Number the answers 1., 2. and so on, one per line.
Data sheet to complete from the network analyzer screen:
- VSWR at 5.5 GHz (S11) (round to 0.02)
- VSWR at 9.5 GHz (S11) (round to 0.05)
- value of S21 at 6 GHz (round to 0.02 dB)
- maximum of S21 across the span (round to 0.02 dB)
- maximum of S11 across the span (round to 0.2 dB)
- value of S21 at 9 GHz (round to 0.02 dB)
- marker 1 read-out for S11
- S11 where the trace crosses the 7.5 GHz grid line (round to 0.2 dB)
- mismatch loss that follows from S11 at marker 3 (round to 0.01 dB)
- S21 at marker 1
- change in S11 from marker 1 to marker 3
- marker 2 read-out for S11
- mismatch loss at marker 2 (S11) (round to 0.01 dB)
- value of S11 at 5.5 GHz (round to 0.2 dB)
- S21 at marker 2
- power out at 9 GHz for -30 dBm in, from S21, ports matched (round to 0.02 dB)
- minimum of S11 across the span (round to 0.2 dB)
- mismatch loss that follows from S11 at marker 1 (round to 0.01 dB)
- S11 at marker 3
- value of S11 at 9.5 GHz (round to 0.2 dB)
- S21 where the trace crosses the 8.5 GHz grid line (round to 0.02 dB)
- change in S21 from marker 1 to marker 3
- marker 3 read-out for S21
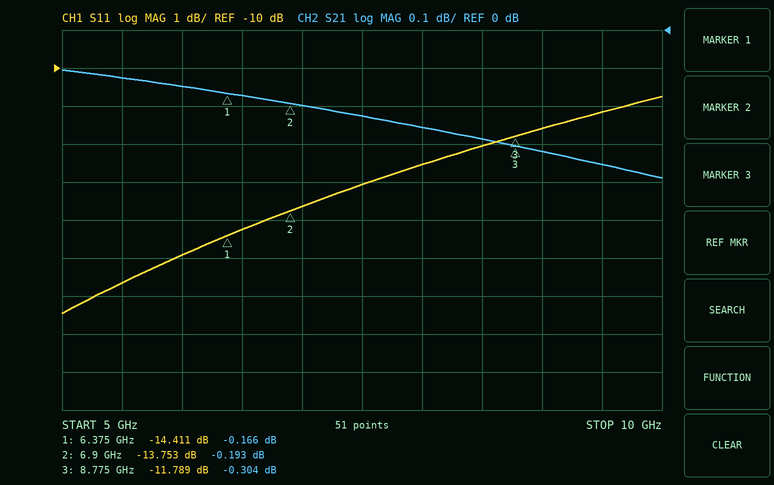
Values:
1. 1.40
2. 1.75
3. -0.14 dB
4. -0.10 dB
5. -10.8 dB
6. -0.32 dB
7. -14.411 dB
8. -13.0 dB
9. 0.30 dB
10. -0.166 dB
11. 2.622 dB
12. -13.753 dB
13. 0.19 dB
14. -15.6 dB
15. -0.193 dB
16. -30.32 dBm
17. -16.4 dB
18. 0.16 dB
19. -11.789 dB
20. -11.2 dB
21. -0.28 dB
22. -0.138 dB
23. -0.304 dB
